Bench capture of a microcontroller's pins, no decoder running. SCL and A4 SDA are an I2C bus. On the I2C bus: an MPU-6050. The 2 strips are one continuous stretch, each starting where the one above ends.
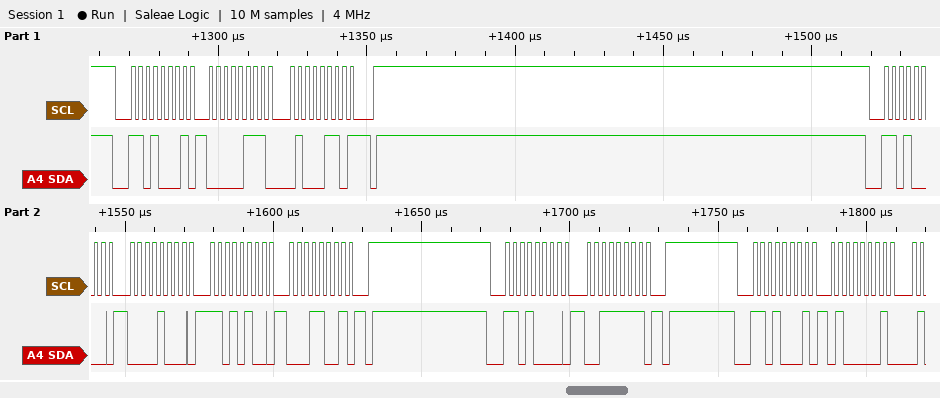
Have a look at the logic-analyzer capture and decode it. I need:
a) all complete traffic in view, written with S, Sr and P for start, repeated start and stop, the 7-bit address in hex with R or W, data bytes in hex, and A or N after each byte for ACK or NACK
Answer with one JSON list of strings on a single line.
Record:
["S 68R A 07 A 46 N P S 68W A 08 A D4 A 19 A P S 68W A 3F A P S 68R A 41 A"]
